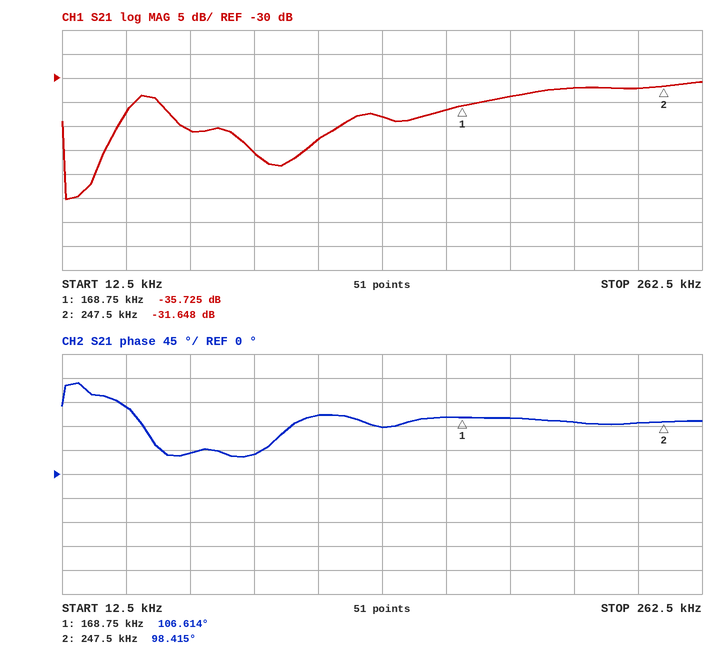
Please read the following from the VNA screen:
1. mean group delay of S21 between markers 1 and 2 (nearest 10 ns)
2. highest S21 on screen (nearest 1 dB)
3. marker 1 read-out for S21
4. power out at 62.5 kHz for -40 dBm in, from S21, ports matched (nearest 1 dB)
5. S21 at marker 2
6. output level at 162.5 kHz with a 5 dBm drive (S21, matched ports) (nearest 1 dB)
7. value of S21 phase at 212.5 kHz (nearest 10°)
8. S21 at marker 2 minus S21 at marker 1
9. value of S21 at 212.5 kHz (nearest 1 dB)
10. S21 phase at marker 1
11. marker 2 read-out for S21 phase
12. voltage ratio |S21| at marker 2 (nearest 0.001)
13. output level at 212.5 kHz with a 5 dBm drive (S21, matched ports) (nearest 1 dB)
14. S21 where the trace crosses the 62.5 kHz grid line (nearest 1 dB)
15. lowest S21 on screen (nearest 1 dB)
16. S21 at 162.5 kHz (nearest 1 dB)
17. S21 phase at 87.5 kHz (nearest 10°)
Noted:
290 ns
-31 dB
-35.725 dB
-81 dBm
-31.648 dB
-32 dBm
100°
4.077 dB
-32 dB
106.614°
98.415°
0.026
-27 dBm
-41 dB
-55 dB
-37 dB
40°
